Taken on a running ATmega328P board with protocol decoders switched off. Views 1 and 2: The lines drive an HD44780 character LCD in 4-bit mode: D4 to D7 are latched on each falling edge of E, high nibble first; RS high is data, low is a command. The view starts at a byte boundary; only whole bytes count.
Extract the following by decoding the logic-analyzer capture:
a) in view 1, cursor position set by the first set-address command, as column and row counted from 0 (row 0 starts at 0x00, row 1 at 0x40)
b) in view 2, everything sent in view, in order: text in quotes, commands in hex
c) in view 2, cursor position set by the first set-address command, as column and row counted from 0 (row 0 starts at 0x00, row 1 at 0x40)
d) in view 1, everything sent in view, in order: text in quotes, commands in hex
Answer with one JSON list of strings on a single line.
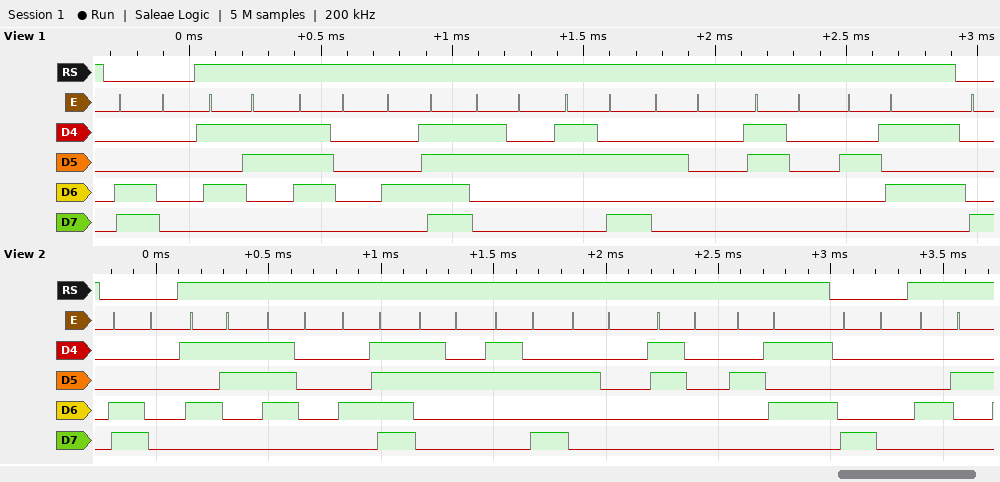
["column 0, row 1", "0xC0 \"SpO2: 0%\" 0x80 \"B\"", "column 0, row 1", "0xC0 \"SpO2: 0%\""]
